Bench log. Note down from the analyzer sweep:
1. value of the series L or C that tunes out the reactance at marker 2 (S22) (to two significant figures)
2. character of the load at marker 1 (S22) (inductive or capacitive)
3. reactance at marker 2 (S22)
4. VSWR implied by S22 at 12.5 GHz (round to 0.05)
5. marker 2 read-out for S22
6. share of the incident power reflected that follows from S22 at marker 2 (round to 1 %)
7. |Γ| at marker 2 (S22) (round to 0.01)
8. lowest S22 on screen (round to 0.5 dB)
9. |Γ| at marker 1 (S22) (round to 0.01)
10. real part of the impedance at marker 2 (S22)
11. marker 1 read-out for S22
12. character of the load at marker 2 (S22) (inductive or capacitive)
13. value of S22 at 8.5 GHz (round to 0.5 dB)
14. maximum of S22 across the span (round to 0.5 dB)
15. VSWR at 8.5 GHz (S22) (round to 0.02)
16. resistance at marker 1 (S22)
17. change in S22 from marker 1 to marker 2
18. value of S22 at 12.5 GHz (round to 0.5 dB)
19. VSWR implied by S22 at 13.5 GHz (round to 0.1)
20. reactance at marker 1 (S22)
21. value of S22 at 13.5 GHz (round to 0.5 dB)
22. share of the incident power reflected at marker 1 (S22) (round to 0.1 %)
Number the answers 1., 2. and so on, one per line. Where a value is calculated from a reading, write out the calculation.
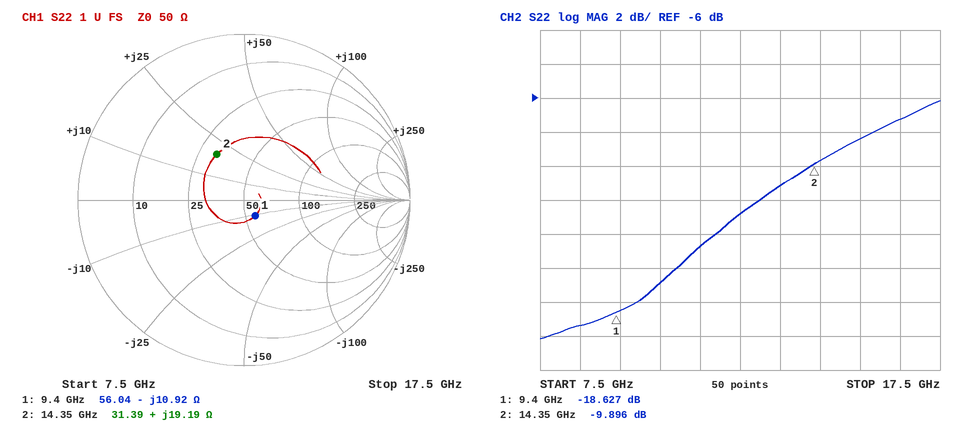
1. C = 1/(2π × 14.35 GHz × 19.19 Ω) ≈ 578 fF, so 580 fF to two significant figures
2. capacitive
3. +19.19 Ω
4. |Γ| = 10^(-13/20) = 0.2239; VSWR = (1 + 0.2239)/(1 − 0.2239) ≈ 1.58, so 1.60 to the nearest 0.05
5. -9.896 dB
6. 10^(-9.896/10) ≈ 10 %
7. 0.32
8. -20.0 dB
9. 0.12
10. 31.39 Ω
11. -18.627 dB
12. inductive
13. -19.5 dB
14. -6.0 dB
15. |Γ| = 10^(-19.5/20) = 0.1059; VSWR = (1 + 0.1059)/(1 − 0.1059) ≈ 1.24
16. 56.04 Ω
17. -9.896 − (-18.627) = 8.731 dB
18. -13.0 dB
19. |Γ| = 10^(-11/20) = 0.2818; VSWR = (1 + 0.2818)/(1 − 0.2818) ≈ 1.8
20. -10.92 Ω
21. -11.0 dB
22. 10^(-18.627/10) ≈ 1.4 %
